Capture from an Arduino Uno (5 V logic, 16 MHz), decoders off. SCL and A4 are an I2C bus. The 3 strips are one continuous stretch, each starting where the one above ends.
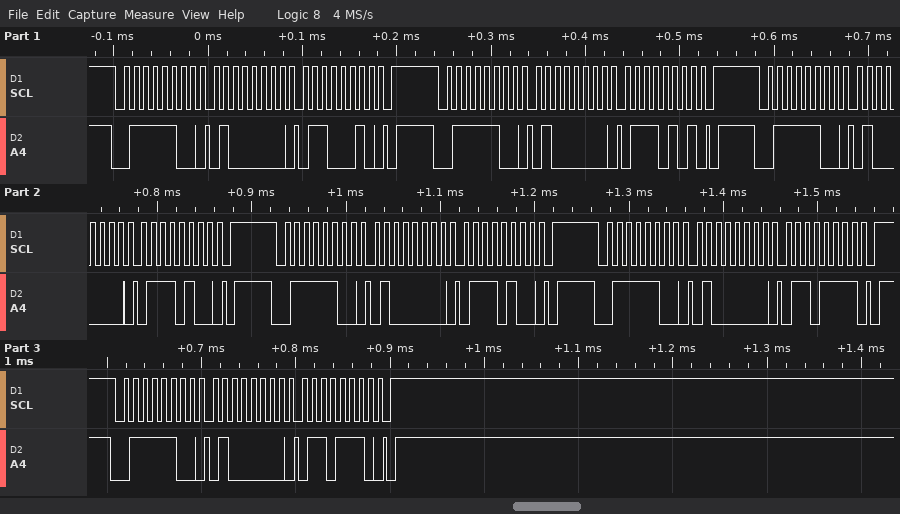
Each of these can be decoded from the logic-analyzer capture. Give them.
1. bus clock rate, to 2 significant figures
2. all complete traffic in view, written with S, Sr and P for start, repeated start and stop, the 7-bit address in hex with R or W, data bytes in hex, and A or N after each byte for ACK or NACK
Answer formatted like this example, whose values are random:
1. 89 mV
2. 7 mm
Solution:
1. 100 kHz
2. S 3EW A 40 A 62 A P S 3EW A 40 A 75 A P S 3EW A 40 A 74 A P S 3EW A 40 A 74 A P S 3EW A 40 A 6F A P S 3EW A 40 A 6E A P
